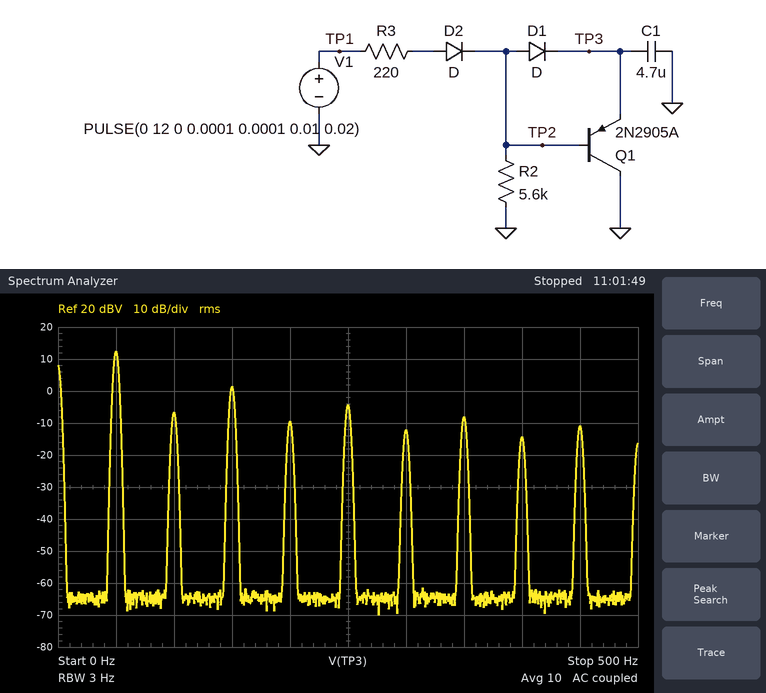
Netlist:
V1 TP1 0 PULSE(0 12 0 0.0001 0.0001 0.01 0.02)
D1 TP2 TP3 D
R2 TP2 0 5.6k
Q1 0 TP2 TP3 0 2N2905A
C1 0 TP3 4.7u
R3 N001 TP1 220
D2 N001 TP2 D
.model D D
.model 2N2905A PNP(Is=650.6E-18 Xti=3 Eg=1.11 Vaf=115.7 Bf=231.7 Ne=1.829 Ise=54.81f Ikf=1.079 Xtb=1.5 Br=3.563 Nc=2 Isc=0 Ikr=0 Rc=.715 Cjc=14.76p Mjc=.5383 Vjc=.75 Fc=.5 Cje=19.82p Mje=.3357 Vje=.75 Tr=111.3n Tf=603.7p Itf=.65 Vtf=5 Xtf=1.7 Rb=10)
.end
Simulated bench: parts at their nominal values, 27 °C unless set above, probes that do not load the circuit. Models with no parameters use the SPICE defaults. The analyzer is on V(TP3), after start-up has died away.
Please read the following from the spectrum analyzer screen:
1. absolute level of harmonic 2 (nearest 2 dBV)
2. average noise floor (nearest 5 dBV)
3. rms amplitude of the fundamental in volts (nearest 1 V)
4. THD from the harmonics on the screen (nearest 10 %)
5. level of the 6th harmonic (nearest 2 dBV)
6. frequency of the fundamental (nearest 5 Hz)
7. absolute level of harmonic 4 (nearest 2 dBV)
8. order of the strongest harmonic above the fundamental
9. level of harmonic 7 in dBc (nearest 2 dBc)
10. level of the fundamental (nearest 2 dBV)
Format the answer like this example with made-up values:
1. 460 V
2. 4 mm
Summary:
1. -6 dBV
2. -65 dBV
3. 4 V
4. 40 %
5. -12 dBV
6. 50 Hz
7. -10 dBV
8. 3
9. -20 dBc
10. 12 dBV
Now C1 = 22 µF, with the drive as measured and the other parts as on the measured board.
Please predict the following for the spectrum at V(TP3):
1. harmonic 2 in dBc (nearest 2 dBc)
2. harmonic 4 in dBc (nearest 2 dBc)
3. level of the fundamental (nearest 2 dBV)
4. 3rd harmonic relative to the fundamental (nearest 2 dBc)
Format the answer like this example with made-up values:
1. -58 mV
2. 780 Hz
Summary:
1. -12 dBc
2. -20 dBc
3. 10 dBV
4. -12 dBc
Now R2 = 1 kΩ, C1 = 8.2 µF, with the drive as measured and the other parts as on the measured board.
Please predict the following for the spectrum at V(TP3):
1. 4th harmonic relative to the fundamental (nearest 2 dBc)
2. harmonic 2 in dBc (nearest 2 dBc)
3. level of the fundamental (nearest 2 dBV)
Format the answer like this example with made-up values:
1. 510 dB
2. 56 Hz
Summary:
1. -20 dBc
2. -16 dBc
3. 10 dBV
